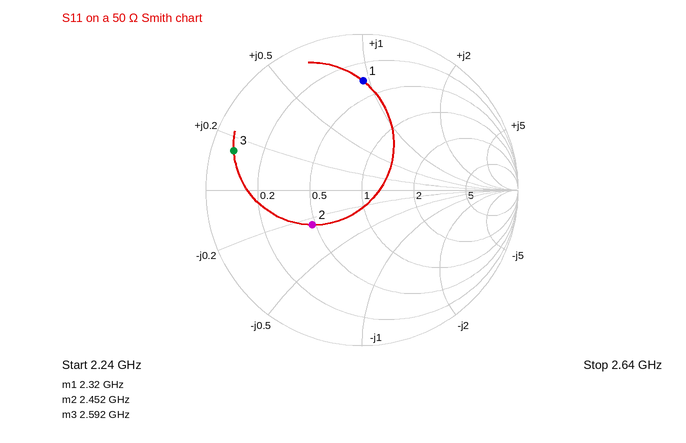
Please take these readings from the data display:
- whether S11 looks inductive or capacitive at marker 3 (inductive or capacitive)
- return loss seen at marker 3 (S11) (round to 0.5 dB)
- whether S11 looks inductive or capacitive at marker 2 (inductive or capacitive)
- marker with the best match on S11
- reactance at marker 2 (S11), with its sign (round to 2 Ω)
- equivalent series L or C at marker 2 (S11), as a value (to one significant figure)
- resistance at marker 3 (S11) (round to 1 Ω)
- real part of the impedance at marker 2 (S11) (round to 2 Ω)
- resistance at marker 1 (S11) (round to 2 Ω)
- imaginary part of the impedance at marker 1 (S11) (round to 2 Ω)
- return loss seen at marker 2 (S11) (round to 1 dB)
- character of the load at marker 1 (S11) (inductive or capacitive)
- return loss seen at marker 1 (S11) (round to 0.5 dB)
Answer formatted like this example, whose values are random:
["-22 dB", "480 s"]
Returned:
["inductive", "1.5 dB", "capacitive", "marker 2", "-12 Ω", "5 pF", "4 Ω", "24 Ω", "18 Ω", "+48 Ω", "8 dB", "inductive", "3.0 dB"]
